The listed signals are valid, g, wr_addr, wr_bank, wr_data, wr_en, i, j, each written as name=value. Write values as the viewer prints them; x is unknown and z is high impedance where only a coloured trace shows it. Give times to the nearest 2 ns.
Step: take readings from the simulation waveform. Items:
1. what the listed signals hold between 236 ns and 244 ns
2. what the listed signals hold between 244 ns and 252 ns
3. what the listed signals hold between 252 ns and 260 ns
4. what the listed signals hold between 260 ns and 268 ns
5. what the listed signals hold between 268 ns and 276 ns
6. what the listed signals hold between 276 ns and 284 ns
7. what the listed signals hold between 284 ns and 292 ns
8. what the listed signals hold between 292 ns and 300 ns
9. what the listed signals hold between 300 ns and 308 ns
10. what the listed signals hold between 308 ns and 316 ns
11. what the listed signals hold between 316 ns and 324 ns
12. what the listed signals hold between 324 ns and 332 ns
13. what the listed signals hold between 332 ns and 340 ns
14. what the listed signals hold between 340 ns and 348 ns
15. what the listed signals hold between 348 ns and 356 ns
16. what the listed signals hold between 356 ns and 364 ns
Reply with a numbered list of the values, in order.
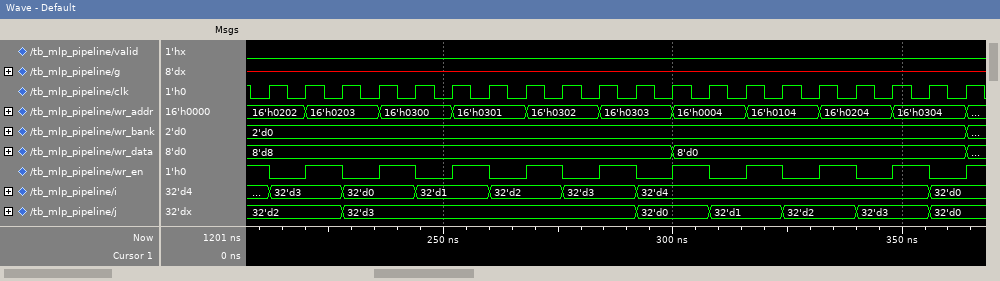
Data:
1. valid=0, g=x, wr_addr=16'h0300, wr_bank=2'd0, wr_data=8'd8, wr_en=1, i=32'd0, j=32'd3
2. valid=0, g=x, wr_addr=16'h0300, wr_bank=2'd0, wr_data=8'd8, wr_en=0, i=32'd1, j=32'd3
3. valid=0, g=x, wr_addr=16'h0301, wr_bank=2'd0, wr_data=8'd8, wr_en=1, i=32'd1, j=32'd3
4. valid=0, g=x, wr_addr=16'h0301, wr_bank=2'd0, wr_data=8'd8, wr_en=0, i=32'd2, j=32'd3
5. valid=0, g=x, wr_addr=16'h0302, wr_bank=2'd0, wr_data=8'd8, wr_en=1, i=32'd2, j=32'd3
6. valid=0, g=x, wr_addr=16'h0302, wr_bank=2'd0, wr_data=8'd8, wr_en=0, i=32'd3, j=32'd3
7. valid=0, g=x, wr_addr=16'h0303, wr_bank=2'd0, wr_data=8'd8, wr_en=1, i=32'd3, j=32'd3
8. valid=0, g=x, wr_addr=16'h0303, wr_bank=2'd0, wr_data=8'd8, wr_en=0, i=32'd4, j=32'd0
9. valid=0, g=x, wr_addr=16'h0004, wr_bank=2'd0, wr_data=8'd0, wr_en=1, i=32'd4, j=32'd0
10. valid=0, g=x, wr_addr=16'h0004, wr_bank=2'd0, wr_data=8'd0, wr_en=0, i=32'd4, j=32'd1
11. valid=0, g=x, wr_addr=16'h0104, wr_bank=2'd0, wr_data=8'd0, wr_en=1, i=32'd4, j=32'd1
12. valid=0, g=x, wr_addr=16'h0104, wr_bank=2'd0, wr_data=8'd0, wr_en=0, i=32'd4, j=32'd2
13. valid=0, g=x, wr_addr=16'h0204, wr_bank=2'd0, wr_data=8'd0, wr_en=1, i=32'd4, j=32'd2
14. valid=0, g=x, wr_addr=16'h0204, wr_bank=2'd0, wr_data=8'd0, wr_en=0, i=32'd4, j=32'd3
15. valid=0, g=x, wr_addr=16'h0304, wr_bank=2'd0, wr_data=8'd0, wr_en=1, i=32'd4, j=32'd3
16. valid=0, g=x, wr_addr=16'h0304, wr_bank=2'd0, wr_data=8'd0, wr_en=0, i=32'd0, j=32'd0
